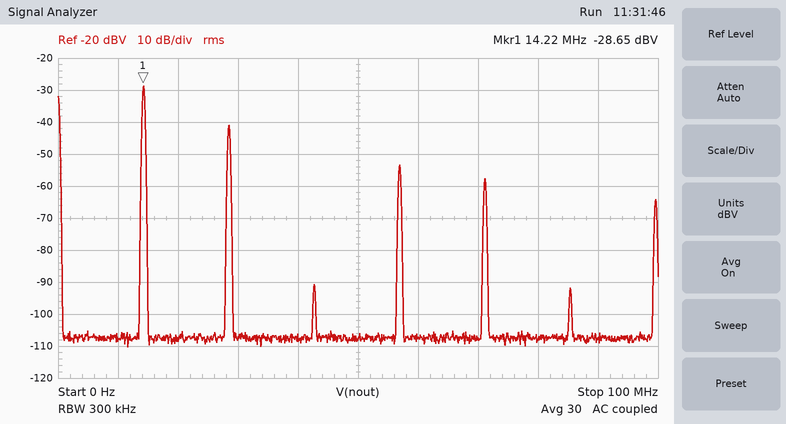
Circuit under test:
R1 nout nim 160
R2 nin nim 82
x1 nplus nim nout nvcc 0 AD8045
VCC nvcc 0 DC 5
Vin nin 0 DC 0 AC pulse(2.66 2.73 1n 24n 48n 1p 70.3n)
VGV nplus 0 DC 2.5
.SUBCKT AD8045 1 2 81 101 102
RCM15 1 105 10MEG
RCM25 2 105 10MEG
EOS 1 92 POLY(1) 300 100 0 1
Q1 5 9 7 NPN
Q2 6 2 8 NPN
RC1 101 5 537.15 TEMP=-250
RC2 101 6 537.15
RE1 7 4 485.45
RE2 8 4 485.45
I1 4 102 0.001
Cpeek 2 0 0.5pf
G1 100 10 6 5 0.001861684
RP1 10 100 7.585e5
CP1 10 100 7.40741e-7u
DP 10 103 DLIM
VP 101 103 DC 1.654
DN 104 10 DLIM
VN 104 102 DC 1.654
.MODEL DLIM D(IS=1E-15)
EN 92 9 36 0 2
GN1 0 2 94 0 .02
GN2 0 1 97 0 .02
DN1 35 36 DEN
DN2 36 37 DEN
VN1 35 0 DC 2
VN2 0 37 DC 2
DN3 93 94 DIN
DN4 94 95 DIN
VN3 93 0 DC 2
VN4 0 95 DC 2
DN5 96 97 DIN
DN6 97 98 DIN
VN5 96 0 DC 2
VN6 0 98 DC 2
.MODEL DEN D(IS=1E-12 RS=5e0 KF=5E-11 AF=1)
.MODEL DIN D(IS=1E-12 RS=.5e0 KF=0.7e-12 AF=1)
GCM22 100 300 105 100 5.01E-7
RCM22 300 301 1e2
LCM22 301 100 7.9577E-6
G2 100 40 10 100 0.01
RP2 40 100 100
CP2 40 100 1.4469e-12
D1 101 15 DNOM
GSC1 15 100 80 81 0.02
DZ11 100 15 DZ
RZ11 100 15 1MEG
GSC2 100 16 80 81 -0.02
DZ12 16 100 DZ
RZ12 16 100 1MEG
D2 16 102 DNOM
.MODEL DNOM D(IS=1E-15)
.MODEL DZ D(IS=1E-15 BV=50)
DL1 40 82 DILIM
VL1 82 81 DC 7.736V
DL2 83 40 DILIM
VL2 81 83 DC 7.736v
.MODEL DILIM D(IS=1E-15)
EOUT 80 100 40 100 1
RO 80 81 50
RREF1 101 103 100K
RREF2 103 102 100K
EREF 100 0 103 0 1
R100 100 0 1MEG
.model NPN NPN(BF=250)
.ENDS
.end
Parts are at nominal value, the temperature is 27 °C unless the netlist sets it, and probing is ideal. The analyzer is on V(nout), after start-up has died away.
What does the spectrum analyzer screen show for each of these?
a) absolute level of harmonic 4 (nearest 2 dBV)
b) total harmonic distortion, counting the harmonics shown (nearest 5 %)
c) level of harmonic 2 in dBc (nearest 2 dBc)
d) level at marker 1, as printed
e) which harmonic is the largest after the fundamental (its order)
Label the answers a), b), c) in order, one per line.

a) -54 dBV
b) 25 %
c) -12 dBc
d) -28.65 dBV
e) 2
